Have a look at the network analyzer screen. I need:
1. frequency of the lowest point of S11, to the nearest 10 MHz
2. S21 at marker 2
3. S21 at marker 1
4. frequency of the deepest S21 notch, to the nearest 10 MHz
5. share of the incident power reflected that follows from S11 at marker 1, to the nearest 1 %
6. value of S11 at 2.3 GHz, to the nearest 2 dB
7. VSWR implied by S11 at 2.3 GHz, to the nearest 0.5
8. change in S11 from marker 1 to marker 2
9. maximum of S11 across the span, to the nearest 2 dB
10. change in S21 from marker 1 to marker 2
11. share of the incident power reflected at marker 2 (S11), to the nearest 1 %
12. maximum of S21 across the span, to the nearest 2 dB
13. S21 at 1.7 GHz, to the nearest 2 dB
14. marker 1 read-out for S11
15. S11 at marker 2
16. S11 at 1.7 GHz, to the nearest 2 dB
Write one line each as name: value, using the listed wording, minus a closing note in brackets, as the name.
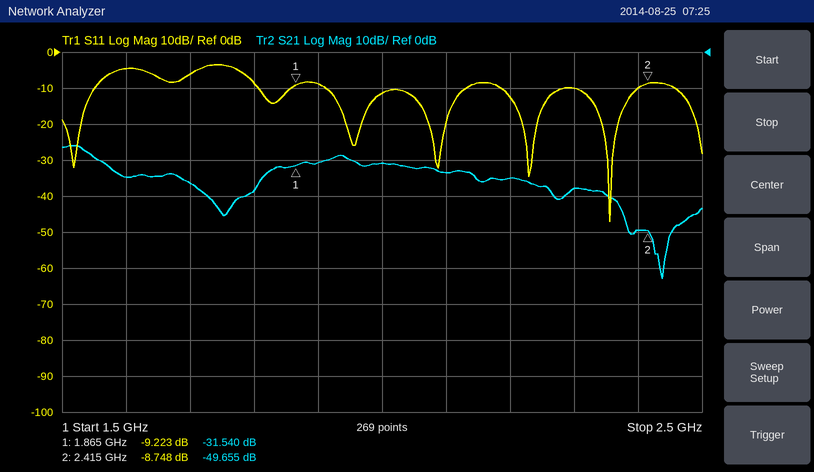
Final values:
frequency of the lowest point of S11, to the nearest 10 MHz: 2.36 GHz
S21 at marker 2: -49.655 dB
S21 at marker 1: -31.540 dB
frequency of the deepest S21 notch, to the nearest 10 MHz: 2.44 GHz
share of the incident power reflected that follows from S11 at marker 1, to the nearest 1 %: 12 %
value of S11 at 2.3 GHz, to the nearest 2 dB: -10 dB
VSWR implied by S11 at 2.3 GHz, to the nearest 0.5: 2.0
change in S11 from marker 1 to marker 2: 0.475 dB
maximum of S11 across the span, to the nearest 2 dB: -4 dB
change in S21 from marker 1 to marker 2: -18.115 dB
share of the incident power reflected at marker 2 (S11), to the nearest 1 %: 13 %
maximum of S21 across the span, to the nearest 2 dB: -26 dB
S21 at 1.7 GHz, to the nearest 2 dB: -36 dB
marker 1 read-out for S11: -9.223 dB
S11 at marker 2: -8.748 dB
S11 at 1.7 GHz, to the nearest 2 dB: -6 dB
